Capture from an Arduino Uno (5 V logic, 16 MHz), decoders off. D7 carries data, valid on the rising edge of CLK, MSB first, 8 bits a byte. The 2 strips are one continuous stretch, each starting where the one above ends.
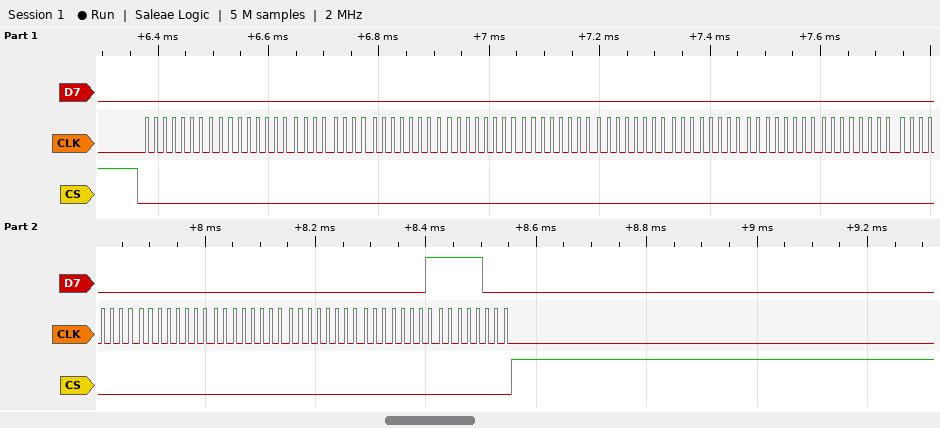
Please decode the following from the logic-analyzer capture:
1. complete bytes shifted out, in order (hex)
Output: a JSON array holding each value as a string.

["00 00 00 00 00 00 00 00 00 00 00 00 00 00 01 F8"]
